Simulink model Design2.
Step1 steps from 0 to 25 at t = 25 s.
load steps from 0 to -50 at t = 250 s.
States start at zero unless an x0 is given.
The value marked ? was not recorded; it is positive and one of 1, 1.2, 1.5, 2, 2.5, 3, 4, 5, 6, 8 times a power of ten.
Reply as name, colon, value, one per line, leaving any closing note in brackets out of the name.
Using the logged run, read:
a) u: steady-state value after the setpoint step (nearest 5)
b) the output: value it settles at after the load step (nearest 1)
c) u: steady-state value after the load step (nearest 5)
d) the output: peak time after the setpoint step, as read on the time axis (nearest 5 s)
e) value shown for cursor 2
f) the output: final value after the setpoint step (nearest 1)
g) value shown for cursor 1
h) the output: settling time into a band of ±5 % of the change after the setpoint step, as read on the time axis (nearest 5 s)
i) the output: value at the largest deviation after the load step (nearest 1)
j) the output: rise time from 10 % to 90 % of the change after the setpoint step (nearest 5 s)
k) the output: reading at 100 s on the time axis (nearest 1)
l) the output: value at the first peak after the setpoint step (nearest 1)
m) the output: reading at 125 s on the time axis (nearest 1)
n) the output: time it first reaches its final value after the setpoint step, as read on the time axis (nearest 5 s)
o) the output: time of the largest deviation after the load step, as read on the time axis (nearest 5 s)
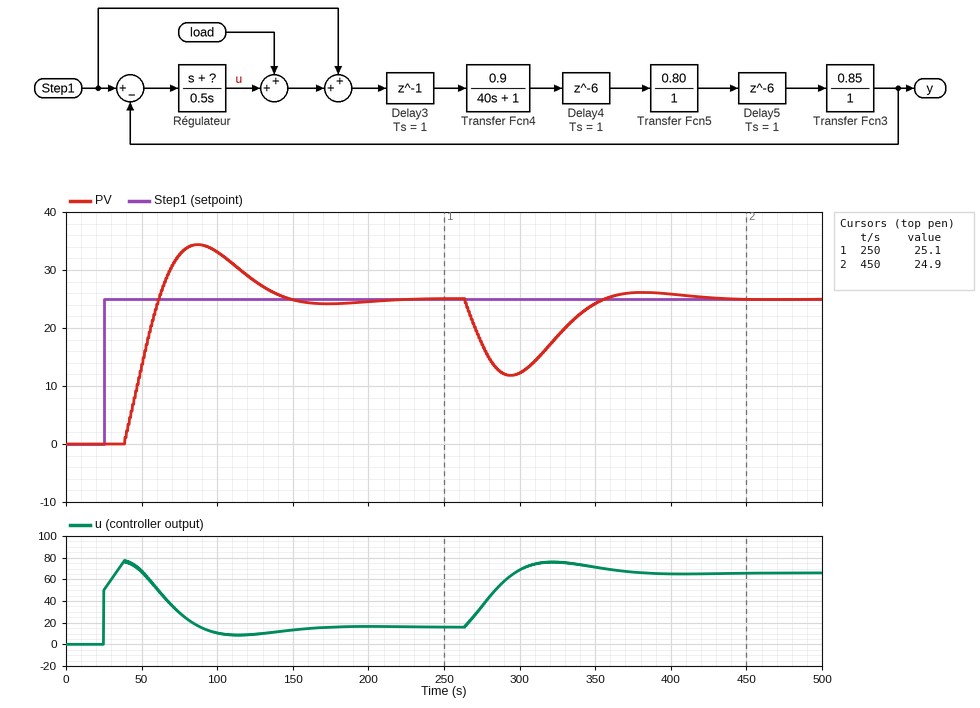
u: steady-state value after the setpoint step: 15
the output: value it settles at after the load step: 25
u: steady-state value after the load step: 65
the output: peak time after the setpoint step, as read on the time axis: 85 s
value shown for cursor 2: 24.9
the output: final value after the setpoint step: 25
value shown for cursor 1: 25.1
the output: settling time into a band of ±5 % of the change after the setpoint step, as read on the time axis: 135 s
the output: value at the largest deviation after the load step: 12
the output: rise time from 10 % to 90 % of the change after the setpoint step: 20 s
the output: reading at 100 s on the time axis: 33
the output: value at the first peak after the setpoint step: 34
the output: reading at 125 s on the time axis: 28
the output: time it first reaches its final value after the setpoint step, as read on the time axis: 60 s
the output: time of the largest deviation after the load step, as read on the time axis: 295 s
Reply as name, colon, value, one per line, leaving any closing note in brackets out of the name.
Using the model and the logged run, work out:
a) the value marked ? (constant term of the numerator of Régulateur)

the value marked ?: 0.04
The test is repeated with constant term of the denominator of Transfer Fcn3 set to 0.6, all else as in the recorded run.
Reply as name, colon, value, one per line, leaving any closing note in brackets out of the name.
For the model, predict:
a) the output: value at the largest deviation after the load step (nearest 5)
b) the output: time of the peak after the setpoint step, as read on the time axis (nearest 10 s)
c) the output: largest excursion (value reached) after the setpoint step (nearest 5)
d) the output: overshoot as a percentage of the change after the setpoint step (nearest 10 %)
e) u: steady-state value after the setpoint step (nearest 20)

the output: value at the largest deviation after the load step: 5
the output: time of the peak after the setpoint step, as read on the time axis: 70 s
the output: largest excursion (value reached) after the setpoint step: 45
the output: overshoot as a percentage of the change after the setpoint step: 80 %
u: steady-state value after the setpoint step: 0
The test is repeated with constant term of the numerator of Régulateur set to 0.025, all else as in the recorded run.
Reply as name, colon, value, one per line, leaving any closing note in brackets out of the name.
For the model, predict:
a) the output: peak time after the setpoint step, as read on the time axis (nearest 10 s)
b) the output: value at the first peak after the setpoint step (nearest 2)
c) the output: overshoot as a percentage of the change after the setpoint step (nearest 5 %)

the output: peak time after the setpoint step, as read on the time axis: 90 s
the output: value at the first peak after the setpoint step: 30
the output: overshoot as a percentage of the change after the setpoint step: 20 %
